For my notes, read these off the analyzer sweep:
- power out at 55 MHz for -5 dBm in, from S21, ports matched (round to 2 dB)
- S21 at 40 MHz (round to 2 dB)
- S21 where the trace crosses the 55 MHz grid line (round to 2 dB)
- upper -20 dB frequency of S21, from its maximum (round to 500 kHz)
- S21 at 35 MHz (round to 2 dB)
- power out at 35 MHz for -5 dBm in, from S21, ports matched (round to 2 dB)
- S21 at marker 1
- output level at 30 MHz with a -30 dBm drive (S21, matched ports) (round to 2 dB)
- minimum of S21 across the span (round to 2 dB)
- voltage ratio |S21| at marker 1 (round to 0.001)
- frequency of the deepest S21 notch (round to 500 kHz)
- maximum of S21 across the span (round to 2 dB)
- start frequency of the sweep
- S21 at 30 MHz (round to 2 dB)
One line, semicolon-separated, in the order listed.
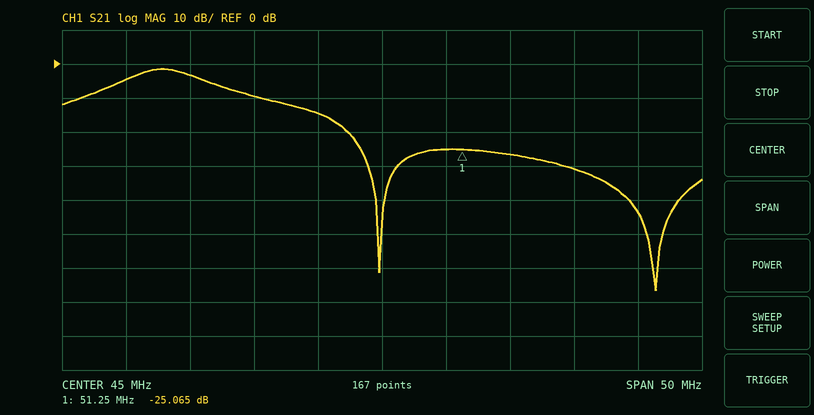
-32 dBm; -14 dB; -26 dB; 42.5 MHz; -10 dB; -14 dBm; -25.065 dB; -34 dBm; -66 dB; 0.056; 66.5 MHz; -2 dB; 20 MHz; -4 dB
